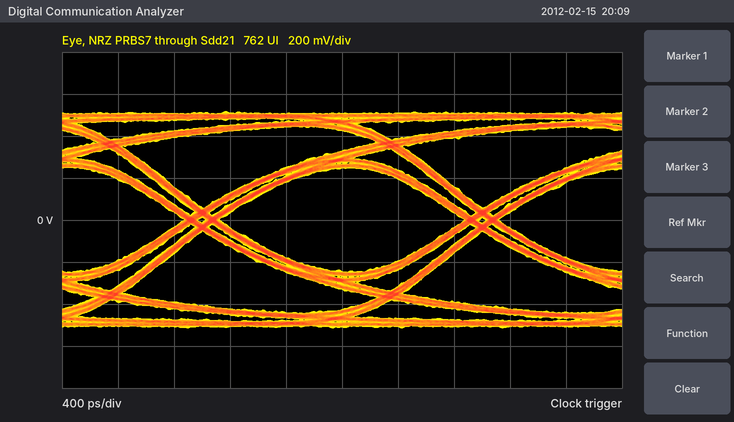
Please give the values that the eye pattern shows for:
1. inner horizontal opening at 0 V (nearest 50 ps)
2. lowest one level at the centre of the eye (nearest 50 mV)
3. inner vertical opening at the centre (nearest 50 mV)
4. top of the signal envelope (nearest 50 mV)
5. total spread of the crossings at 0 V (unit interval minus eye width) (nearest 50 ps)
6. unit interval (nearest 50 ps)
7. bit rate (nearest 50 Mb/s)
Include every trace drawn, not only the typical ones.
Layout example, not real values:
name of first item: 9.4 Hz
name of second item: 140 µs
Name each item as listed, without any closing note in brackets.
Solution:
inner horizontal opening at 0 V: 1.75 ns
lowest one level at the centre of the eye: 250 mV
inner vertical opening at the centre: 500 mV
top of the signal envelope: 500 mV
total spread of the crossings at 0 V (unit interval minus eye width): 250 ps
unit interval: 2.00 ns
bit rate: 500 Mb/s
